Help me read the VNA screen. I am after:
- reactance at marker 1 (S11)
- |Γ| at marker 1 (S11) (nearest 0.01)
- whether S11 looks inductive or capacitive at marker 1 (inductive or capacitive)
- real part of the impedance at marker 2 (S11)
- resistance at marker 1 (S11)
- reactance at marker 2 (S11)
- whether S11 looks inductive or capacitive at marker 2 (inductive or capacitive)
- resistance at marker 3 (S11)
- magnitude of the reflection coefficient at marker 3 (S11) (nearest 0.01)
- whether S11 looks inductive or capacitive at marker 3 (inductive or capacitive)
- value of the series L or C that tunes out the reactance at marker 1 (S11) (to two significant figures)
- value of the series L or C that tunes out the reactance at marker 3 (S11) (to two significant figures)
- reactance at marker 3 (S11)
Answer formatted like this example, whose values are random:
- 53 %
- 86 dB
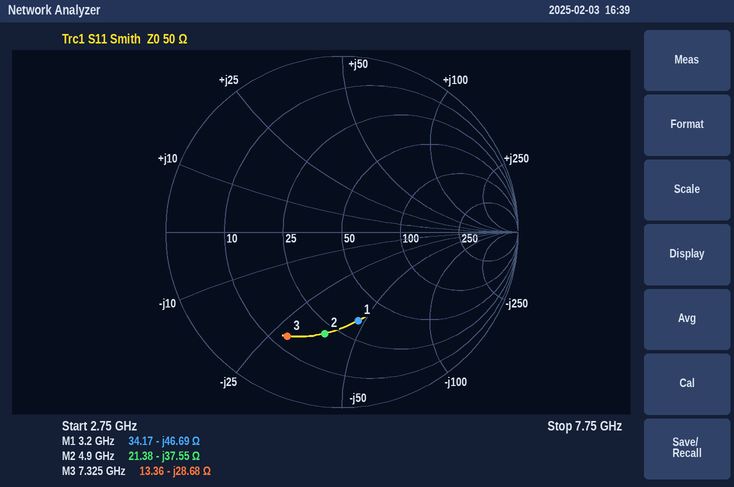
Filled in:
- -46.69 Ω
- 0.51
- capacitive
- 21.38 Ω
- 34.17 Ω
- -37.55 Ω
- capacitive
- 13.36 Ω
- 0.67
- capacitive
- 2.3 nH
- 620 pH
- -28.68 Ω
